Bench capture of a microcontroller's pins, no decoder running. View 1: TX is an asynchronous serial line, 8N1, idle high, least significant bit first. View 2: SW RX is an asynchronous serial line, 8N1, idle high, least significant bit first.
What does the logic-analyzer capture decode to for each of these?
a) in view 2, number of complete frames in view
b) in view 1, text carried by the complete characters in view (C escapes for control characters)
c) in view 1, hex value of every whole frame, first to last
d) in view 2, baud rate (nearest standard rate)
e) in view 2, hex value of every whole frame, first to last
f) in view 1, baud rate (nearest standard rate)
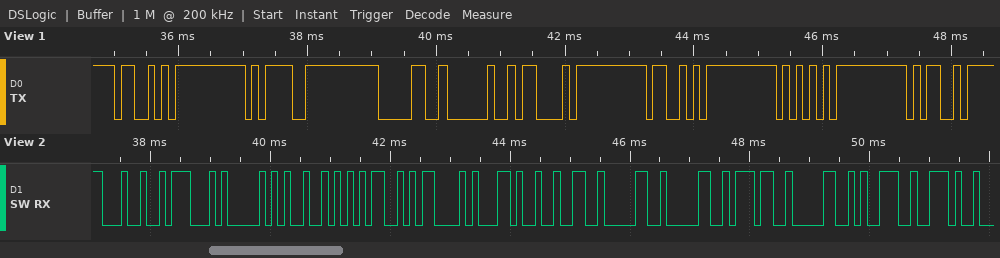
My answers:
14
"S=0 CSUM"
53 3D 30 20 43 53 55 4D
9600 baud
0x24 0x47 0x50 0x52 0x4D 0x43 0x2C 0x32 0x30 0x30 0x37 0x30 0x39 0x2E
9600 baud
